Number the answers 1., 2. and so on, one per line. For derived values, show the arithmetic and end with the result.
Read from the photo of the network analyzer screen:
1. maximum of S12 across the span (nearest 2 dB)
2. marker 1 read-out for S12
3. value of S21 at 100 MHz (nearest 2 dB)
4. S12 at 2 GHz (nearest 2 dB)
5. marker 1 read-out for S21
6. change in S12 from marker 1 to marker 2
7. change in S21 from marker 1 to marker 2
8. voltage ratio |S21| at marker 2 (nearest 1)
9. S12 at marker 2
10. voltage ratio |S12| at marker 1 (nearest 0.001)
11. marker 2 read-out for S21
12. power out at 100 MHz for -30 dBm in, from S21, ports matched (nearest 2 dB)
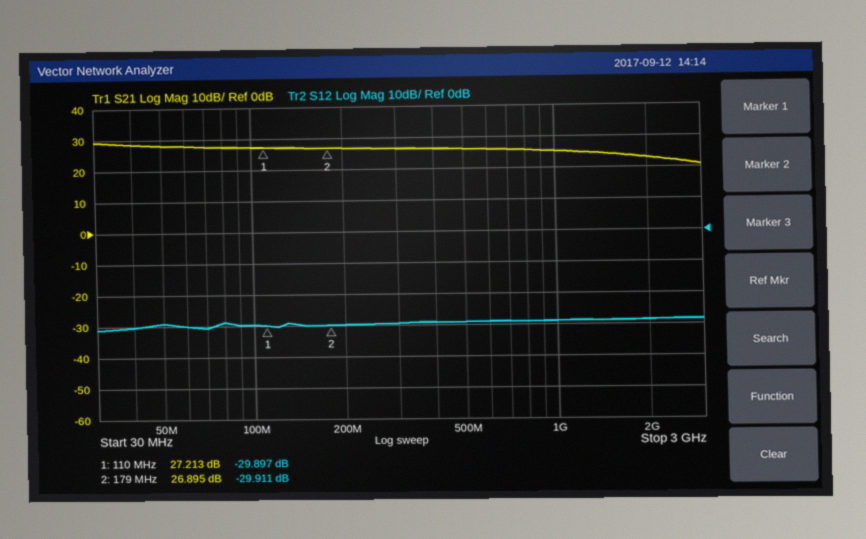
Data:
1. -28 dB
2. -29.897 dB
3. 28 dB
4. -28 dB
5. 27.213 dB
6. -29.911 − (-29.897) = -0.014 dB
7. 26.895 − (27.213) = -0.318 dB
8. 10^(26.895/20) ≈ 22
9. -29.911 dB
10. 10^(-29.897/20) ≈ 0.032
11. 26.895 dB
12. -30 dBm + (28 dB) = -2 dBm
